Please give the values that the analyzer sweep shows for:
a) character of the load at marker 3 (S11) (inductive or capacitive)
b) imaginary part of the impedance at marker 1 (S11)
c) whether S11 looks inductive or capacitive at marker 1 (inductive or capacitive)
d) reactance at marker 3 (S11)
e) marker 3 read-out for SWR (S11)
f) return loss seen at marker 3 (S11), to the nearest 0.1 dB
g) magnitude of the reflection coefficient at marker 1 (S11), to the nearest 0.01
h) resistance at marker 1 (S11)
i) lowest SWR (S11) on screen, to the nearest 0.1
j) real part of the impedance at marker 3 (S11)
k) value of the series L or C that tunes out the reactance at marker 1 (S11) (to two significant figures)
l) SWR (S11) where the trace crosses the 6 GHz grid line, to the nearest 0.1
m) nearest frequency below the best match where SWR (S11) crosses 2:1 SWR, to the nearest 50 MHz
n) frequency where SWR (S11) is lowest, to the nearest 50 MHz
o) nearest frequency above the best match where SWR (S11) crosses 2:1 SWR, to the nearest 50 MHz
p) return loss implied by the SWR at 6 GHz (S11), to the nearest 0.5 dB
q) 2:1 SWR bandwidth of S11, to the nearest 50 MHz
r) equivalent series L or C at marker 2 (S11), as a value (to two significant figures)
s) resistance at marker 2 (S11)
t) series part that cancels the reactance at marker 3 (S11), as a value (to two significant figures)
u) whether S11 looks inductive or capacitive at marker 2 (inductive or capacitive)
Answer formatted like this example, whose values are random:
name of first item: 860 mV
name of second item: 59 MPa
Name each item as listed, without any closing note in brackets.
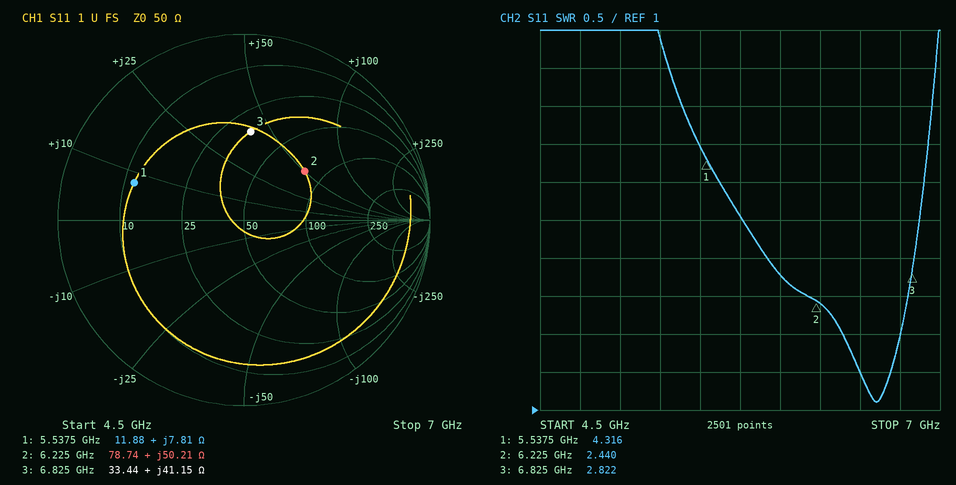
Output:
character of the load at marker 3 (S11): inductive
imaginary part of the impedance at marker 1: +7.81 Ω
whether S11 looks inductive or capacitive at marker 1: inductive
reactance at marker 3: +41.15 Ω
marker 3 read-out for SWR: 2.822
return loss seen at marker 3 (S11), to the nearest 0.1 dB: 6.4 dB
magnitude of the reflection coefficient at marker 1 (S11), to the nearest 0.01: 0.62
resistance at marker 1: 11.88 Ω
lowest SWR (S11) on screen, to the nearest 0.1: 1.1
real part of the impedance at marker 3: 33.44 Ω
value of the series L or C that tunes out the reactance at marker 1 (S11): 3.7 pF
SWR (S11) where the trace crosses the 6 GHz grid line, to the nearest 0.1: 2.8
nearest frequency below the best match where SWR (S11) crosses 2:1 SWR, to the nearest 50 MHz: 6.40 GHz
frequency where SWR (S11) is lowest, to the nearest 50 MHz: 6.60 GHz
nearest frequency above the best match where SWR (S11) crosses 2:1 SWR, to the nearest 50 MHz: 6.75 GHz
return loss implied by the SWR at 6 GHz (S11), to the nearest 0.5 dB: 6.5 dB
2:1 SWR bandwidth of S11, to the nearest 50 MHz: 350 MHz
equivalent series L or C at marker 2 (S11), as a value: 1.3 nH
resistance at marker 2: 78.74 Ω
series part that cancels the reactance at marker 3 (S11), as a value: 570 fF
whether S11 looks inductive or capacitive at marker 2: inductive
